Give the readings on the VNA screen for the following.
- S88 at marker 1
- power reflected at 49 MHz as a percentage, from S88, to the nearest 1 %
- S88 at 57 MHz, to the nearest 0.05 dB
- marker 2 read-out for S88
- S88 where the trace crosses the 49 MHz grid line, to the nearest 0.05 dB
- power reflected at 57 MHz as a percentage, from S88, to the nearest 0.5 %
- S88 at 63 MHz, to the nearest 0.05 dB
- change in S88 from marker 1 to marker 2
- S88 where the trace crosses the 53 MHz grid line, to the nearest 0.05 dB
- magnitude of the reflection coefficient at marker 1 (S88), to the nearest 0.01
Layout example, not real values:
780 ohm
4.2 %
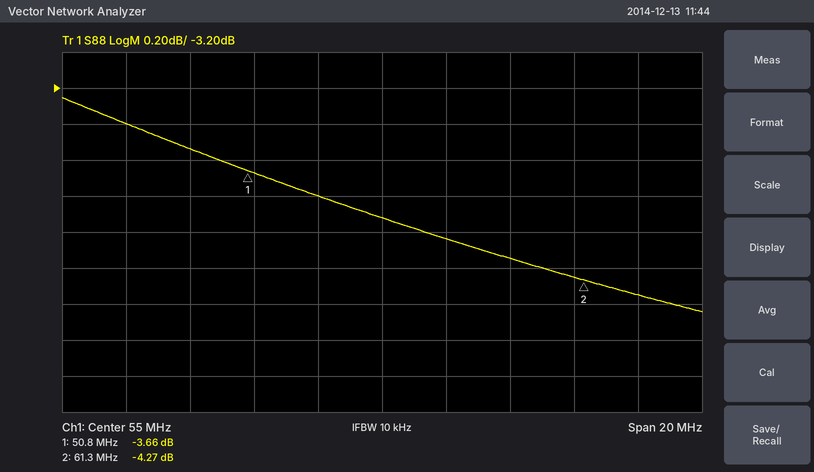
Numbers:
-3.66 dB
44 %
-4.05 dB
-4.27 dB
-3.55 dB
39.5 %
-4.35 dB
-0.61 dB
-3.80 dB
0.66
